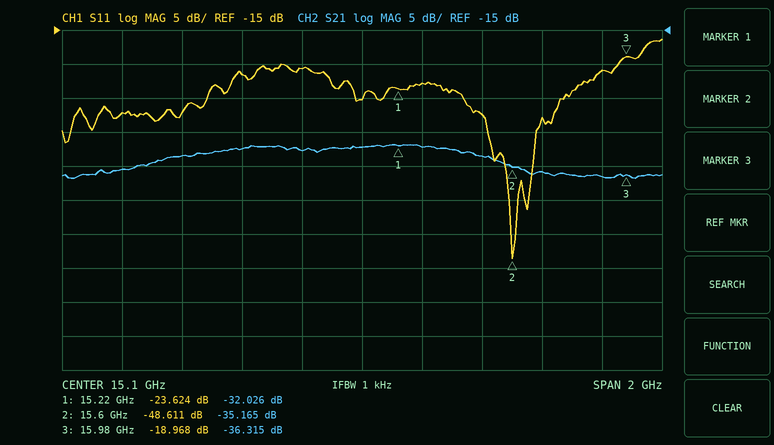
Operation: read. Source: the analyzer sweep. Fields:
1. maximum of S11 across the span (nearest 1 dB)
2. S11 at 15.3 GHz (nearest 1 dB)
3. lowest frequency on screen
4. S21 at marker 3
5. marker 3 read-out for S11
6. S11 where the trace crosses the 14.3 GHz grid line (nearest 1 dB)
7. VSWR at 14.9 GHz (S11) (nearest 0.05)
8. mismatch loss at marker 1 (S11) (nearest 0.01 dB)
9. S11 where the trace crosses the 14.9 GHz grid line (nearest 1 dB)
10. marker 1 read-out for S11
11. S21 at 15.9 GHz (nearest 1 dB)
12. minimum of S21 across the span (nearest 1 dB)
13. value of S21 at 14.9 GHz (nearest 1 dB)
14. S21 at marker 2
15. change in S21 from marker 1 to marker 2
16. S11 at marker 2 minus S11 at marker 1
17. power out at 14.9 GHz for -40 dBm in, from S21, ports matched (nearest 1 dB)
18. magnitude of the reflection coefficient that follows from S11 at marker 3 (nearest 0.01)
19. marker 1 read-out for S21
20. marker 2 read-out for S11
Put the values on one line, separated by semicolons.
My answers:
-16 dB; -23 dB; 14.1 GHz; -36.315 dB; -18.968 dB; -27 dB; 1.20; 0.02 dB; -21 dB; -23.624 dB; -37 dB; -37 dB; -33 dB; -35.165 dB; -3.139 dB; -24.987 dB; -73 dBm; 0.11; -32.026 dB; -48.611 dB
